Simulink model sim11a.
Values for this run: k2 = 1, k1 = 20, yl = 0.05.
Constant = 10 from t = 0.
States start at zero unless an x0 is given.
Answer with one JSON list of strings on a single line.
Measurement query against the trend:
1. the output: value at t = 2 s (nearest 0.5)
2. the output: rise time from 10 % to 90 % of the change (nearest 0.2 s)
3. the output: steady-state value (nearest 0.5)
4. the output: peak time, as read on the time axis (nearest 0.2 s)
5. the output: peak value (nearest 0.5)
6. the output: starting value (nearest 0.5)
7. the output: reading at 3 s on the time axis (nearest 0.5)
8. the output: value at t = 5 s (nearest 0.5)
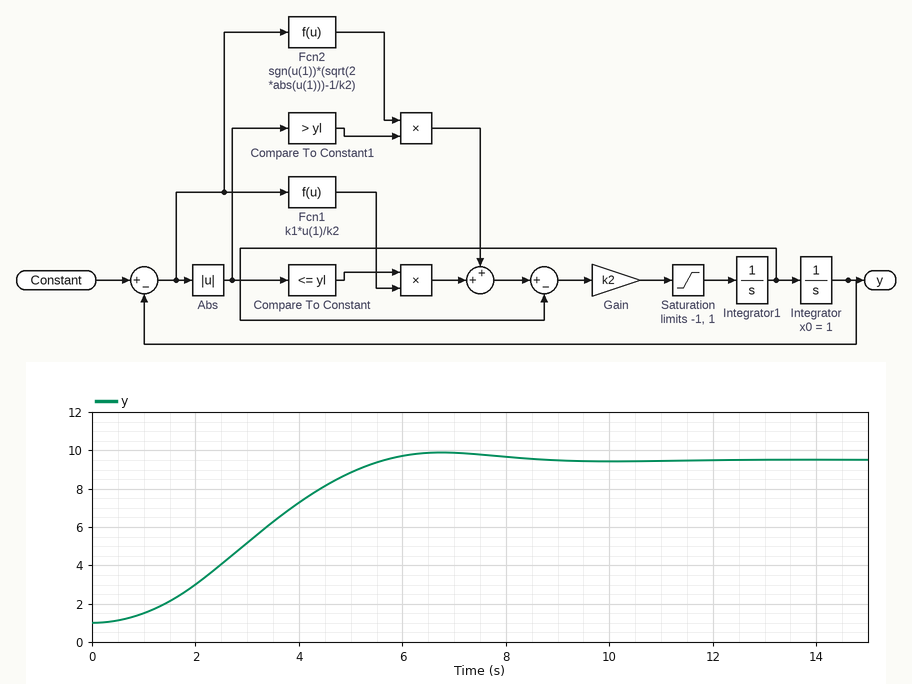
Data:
["3.0", "3.6 s", "9.5", "6.8 s", "10.0", "1.0", "5.0", "9.0"]
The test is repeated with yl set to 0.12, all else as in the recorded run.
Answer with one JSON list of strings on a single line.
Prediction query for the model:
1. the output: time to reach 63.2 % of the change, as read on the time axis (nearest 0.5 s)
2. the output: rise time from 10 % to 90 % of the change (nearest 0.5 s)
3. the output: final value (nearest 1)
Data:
["3.5 s", "4.0 s", "10"]
